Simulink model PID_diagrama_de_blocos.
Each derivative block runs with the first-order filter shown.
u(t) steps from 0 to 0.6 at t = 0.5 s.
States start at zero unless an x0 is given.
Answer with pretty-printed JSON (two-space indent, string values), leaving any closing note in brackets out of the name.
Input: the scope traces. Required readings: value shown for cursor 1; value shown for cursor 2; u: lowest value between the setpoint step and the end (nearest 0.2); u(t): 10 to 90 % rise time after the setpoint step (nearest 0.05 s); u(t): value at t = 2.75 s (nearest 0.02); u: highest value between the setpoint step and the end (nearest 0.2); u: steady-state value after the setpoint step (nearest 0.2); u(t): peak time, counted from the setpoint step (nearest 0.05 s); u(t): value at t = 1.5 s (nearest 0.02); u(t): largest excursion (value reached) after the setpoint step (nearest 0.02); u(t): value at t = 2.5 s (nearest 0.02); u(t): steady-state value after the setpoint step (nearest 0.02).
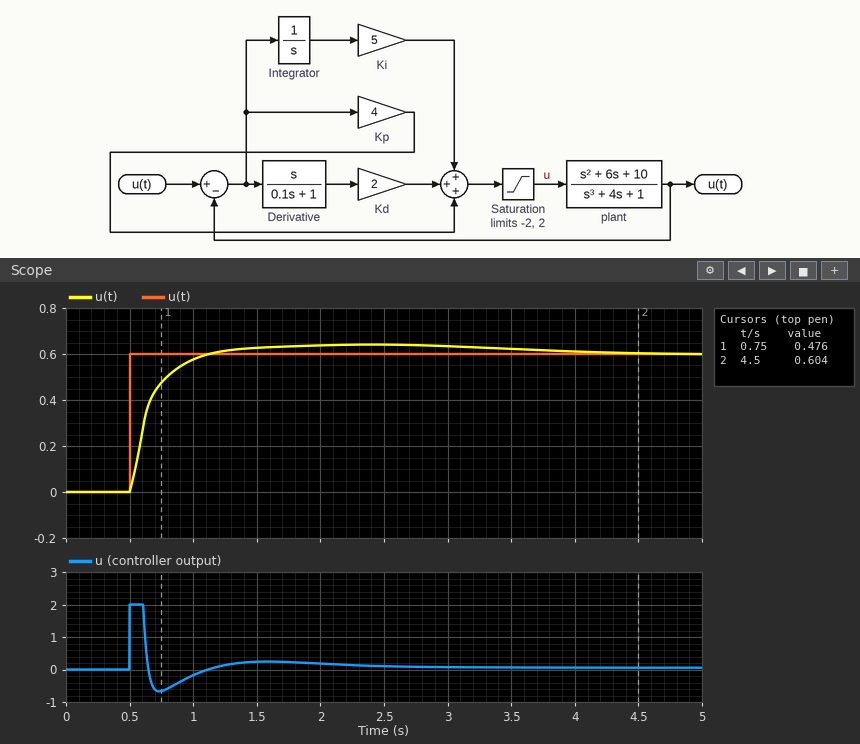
{
  "value shown for cursor 1": "0.476",
  "value shown for cursor 2": "0.604",
  "u: lowest value between the setpoint step and the end": "-0.6",
  "u(t): 10 to 90 % rise time after the setpoint step": "0.35 s",
  "u(t): value at t = 2.75 s": "0.64",
  "u: highest value between the setpoint step and the end": "2.0",
  "u: steady-state value after the setpoint step": "0.0",
  "u(t): peak time, counted from the setpoint step": "1.90 s",
  "u(t): value at t = 1.5 s": "0.62",
  "u(t): largest excursion (value reached) after the setpoint step": "0.64",
  "u(t): value at t = 2.5 s": "0.64",
  "u(t): steady-state value after the setpoint step": "0.60"
}
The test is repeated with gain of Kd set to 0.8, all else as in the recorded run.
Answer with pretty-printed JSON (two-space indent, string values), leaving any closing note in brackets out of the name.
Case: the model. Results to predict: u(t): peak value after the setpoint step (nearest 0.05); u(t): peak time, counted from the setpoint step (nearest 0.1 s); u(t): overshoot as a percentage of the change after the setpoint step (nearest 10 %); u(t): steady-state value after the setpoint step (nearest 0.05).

{
  "u(t): peak value after the setpoint step": "0.70",
  "u(t): peak time, counted from the setpoint step": "0.5 s",
  "u(t): overshoot as a percentage of the change after the setpoint step": "20 %",
  "u(t): steady-state value after the setpoint step": "0.60"
}
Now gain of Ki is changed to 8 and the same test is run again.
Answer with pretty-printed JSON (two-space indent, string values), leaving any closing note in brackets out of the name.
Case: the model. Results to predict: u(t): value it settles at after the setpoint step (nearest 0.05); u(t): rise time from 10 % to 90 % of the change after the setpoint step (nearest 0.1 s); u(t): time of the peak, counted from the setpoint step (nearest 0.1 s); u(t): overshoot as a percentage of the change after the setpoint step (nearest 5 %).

{
  "u(t): value it settles at after the setpoint step": "0.60",
  "u(t): rise time from 10 % to 90 % of the change after the setpoint step": "0.3 s",
  "u(t): time of the peak, counted from the setpoint step": "1.0 s",
  "u(t): overshoot as a percentage of the change after the setpoint step": "10 %"
}
